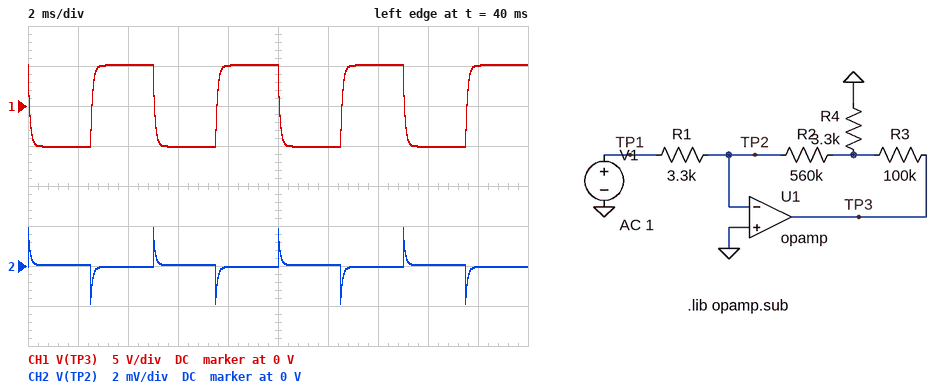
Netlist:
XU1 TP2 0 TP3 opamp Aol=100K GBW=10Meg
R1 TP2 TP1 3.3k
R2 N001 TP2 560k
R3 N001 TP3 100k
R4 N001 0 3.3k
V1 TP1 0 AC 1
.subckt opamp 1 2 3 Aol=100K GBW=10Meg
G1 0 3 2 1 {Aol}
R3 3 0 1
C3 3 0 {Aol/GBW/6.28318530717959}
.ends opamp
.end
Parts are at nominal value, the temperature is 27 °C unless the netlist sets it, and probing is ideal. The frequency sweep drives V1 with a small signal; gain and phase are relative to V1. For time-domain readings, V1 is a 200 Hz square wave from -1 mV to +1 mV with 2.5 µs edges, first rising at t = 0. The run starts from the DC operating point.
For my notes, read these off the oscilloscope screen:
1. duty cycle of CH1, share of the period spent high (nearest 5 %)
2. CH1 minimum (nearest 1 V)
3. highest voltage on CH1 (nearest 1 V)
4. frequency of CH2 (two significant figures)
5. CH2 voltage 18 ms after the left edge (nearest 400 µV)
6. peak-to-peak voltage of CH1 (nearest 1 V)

50 %
-5 V
5 V
200 Hz
0 V
10 V
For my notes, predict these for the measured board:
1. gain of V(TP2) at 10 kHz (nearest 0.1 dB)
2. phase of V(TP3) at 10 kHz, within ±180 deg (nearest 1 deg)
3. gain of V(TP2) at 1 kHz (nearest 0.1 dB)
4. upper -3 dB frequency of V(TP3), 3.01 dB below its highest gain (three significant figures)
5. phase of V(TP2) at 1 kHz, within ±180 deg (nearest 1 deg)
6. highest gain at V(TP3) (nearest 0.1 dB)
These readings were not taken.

-0.2 dB
101 deg
-6.9 dB
1.96 kHz
57 deg
74.1 dB
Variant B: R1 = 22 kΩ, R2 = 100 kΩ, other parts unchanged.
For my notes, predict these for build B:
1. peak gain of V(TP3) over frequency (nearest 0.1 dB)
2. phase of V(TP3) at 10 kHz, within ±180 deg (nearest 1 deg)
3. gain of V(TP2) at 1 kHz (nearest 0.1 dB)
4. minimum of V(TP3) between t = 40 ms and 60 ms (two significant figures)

43.3 dB
170 deg
-36.6 dB
-150 mV
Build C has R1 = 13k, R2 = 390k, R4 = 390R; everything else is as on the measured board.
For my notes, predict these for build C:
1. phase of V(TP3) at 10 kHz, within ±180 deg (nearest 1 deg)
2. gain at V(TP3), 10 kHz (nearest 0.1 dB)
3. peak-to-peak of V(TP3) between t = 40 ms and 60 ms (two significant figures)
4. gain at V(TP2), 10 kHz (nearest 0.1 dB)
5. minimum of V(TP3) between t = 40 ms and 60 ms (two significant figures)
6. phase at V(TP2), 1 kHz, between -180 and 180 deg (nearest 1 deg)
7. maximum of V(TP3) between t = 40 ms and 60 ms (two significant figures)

98 deg
59.6 dB
14 V
-0.4 dB
-7.2 V
48 deg
7.2 V
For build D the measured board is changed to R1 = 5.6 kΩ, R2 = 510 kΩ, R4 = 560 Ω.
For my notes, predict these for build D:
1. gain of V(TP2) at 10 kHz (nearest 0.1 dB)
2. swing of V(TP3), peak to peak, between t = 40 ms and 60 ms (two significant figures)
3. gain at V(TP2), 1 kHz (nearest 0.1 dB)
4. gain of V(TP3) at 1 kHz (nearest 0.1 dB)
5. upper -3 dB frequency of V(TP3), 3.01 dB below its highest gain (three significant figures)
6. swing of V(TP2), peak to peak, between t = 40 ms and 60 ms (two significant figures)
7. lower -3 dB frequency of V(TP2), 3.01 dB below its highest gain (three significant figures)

-0.1 dB
28 V
-1.8 dB
78.2 dB
704 Hz
3.7 mV
690 Hz
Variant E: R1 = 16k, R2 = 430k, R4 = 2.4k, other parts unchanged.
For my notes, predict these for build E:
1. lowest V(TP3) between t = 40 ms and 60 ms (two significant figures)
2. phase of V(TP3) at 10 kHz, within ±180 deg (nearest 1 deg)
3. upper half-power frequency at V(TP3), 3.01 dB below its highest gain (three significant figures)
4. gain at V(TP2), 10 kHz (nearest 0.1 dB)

-1.1 V
130 deg
8.46 kHz
-2.7 dB
